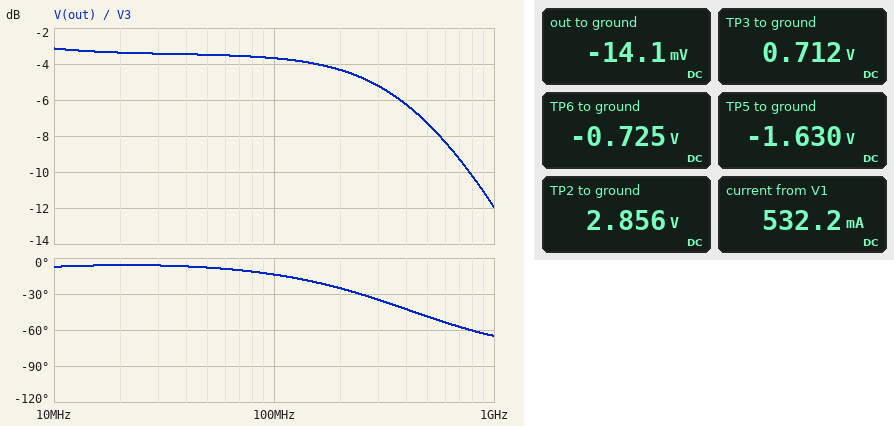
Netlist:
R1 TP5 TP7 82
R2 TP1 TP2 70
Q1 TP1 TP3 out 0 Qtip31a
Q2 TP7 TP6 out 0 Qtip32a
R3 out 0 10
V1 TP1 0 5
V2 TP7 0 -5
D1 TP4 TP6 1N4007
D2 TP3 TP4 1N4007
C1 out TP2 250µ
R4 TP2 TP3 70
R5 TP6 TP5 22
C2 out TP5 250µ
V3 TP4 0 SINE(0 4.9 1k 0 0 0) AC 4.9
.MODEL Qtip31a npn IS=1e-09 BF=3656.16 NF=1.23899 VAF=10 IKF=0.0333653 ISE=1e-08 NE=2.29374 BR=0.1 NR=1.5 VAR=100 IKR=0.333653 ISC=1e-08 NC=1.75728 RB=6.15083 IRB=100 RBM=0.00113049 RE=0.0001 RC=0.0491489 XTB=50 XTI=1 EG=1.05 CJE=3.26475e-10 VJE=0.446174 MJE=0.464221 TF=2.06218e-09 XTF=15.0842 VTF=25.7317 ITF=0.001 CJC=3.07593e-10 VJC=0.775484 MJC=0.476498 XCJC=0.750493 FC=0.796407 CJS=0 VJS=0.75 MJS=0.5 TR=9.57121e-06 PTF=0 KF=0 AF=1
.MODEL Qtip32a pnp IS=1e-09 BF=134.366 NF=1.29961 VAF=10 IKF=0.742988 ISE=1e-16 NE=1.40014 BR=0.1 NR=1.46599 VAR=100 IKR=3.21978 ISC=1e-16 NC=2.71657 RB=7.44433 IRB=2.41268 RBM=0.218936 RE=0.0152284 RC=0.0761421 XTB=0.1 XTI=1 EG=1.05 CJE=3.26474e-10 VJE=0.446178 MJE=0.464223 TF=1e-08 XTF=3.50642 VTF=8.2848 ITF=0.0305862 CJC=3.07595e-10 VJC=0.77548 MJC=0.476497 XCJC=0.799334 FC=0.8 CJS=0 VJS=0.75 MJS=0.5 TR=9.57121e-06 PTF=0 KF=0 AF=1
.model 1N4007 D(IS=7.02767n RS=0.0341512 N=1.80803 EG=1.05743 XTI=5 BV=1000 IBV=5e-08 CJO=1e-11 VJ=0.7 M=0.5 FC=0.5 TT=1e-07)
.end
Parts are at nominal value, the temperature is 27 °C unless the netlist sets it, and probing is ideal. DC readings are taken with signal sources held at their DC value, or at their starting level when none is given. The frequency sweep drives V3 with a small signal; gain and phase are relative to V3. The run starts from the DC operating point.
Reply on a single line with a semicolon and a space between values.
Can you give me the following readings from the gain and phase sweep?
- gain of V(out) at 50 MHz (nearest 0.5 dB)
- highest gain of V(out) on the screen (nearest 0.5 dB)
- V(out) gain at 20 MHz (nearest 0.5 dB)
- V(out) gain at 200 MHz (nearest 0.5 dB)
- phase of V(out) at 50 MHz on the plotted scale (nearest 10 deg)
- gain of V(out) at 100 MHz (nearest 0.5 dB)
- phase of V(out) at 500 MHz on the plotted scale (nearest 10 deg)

-3.5 dB; -3.0 dB; -3.5 dB; -4.5 dB; -10 deg; -3.5 dB; -50 deg
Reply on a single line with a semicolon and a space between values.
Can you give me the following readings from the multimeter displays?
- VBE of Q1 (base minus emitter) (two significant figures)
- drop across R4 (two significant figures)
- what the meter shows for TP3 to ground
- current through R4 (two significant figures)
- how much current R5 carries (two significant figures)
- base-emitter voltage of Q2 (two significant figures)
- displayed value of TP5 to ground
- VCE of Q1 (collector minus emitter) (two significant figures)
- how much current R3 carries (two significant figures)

730 mV; 2.1 V; 0.712 V; 31 mA; 41 mA; -710 mV; -1.630 V; 5.0 V; 1.4 mA
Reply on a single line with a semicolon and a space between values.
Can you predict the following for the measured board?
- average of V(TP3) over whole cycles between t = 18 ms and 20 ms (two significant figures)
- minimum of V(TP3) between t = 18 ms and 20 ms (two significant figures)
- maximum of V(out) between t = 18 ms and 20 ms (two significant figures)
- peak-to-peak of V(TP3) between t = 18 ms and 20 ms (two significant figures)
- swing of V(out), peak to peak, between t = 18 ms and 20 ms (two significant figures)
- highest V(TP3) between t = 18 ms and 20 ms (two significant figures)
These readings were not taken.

710 mV; -4.2 V; 4.7 V; 9.8 V; 9.5 V; 5.6 V
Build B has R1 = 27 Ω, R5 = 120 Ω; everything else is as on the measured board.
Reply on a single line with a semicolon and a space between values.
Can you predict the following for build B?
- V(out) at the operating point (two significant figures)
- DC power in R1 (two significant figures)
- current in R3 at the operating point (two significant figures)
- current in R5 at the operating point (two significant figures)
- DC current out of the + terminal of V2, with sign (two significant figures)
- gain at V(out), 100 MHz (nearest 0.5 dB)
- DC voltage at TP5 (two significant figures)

-5.4 mV; 23 mW; 540 µA; 29 mA; -480 mA; -4.5 dB; -4.2 V
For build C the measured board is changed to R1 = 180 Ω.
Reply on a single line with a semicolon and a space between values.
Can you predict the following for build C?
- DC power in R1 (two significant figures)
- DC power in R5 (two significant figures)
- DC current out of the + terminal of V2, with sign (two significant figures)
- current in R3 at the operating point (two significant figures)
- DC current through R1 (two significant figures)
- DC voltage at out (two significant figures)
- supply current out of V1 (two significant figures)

82 mW; 10 mW; -430 mA; 280 µA; 21 mA; 2.8 mV; 440 mA
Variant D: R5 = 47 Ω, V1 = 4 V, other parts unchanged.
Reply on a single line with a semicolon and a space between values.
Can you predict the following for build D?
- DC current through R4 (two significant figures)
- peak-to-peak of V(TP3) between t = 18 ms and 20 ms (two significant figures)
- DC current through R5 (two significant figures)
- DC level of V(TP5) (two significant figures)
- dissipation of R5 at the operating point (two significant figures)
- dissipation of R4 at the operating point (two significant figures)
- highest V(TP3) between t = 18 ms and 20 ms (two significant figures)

24 mA; 8.9 V; 33 mA; -2.3 V; 52 mW; 39 mW; 4.7 V
